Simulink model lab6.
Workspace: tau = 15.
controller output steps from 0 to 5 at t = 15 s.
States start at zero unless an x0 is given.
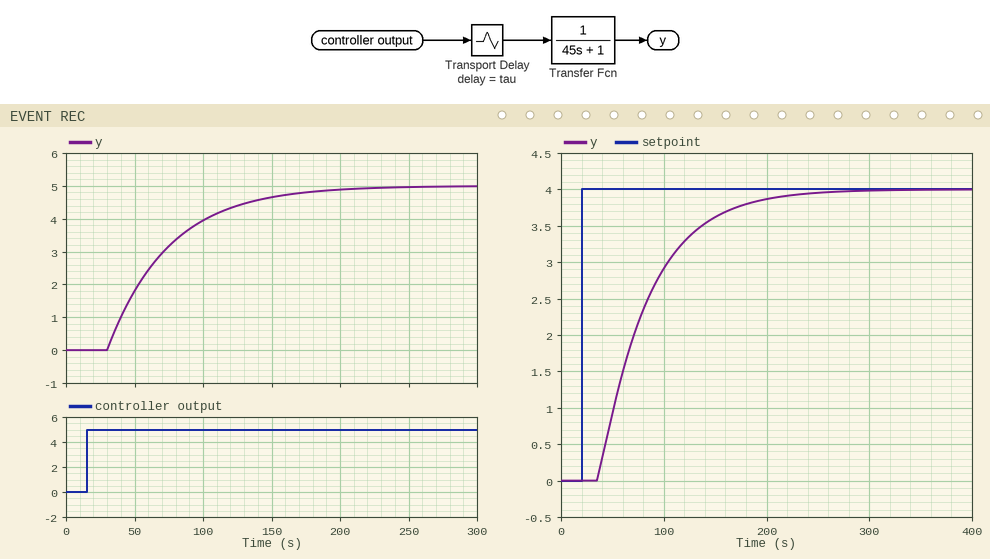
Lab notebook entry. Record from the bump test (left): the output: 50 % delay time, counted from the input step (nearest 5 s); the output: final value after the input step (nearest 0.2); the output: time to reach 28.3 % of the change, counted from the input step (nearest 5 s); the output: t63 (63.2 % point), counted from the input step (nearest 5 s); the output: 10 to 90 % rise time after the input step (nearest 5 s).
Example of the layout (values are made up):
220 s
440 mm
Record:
45 s
5.0
30 s
60 s
100 s
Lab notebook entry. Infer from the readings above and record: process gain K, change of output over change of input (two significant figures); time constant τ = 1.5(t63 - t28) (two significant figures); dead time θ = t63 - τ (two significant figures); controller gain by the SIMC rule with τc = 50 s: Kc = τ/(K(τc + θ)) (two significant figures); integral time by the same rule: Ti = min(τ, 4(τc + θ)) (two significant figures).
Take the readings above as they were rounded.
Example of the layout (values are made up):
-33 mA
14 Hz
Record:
1.0
45 s
15 s
0.69
45 s
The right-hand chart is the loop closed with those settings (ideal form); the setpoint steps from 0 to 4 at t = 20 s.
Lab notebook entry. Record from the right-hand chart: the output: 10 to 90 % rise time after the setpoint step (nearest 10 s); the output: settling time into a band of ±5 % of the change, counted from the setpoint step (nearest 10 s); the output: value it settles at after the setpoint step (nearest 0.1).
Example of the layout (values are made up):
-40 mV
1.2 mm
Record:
110 s
160 s
4.0
